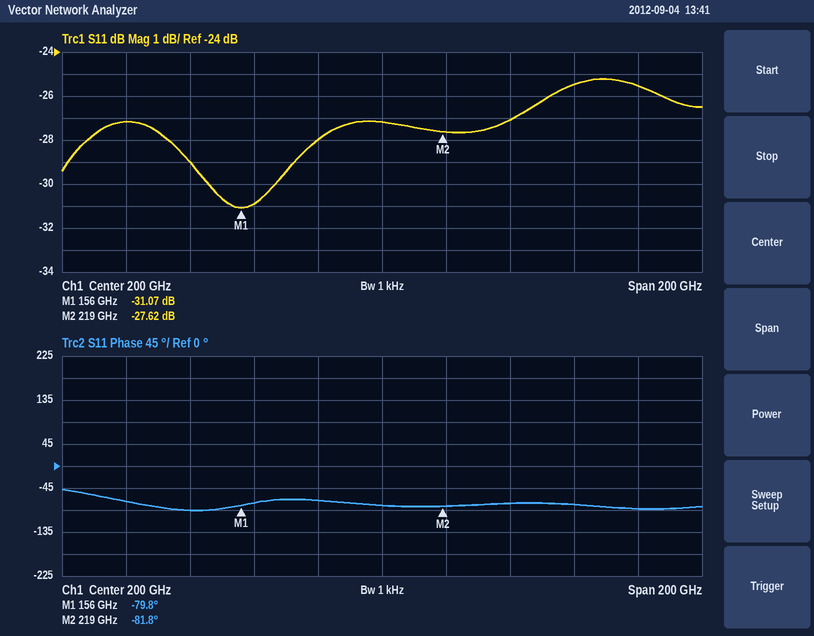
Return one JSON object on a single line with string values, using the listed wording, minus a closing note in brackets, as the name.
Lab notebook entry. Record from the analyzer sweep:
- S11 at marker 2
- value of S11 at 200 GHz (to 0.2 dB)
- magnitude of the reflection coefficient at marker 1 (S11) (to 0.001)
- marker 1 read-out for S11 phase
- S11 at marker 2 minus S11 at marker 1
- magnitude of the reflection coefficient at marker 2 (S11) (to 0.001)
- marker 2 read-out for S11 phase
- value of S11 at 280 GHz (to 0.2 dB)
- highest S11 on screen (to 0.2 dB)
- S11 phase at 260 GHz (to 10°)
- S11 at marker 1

{"S11 at marker 2": "-27.62 dB", "value of S11 at 200 GHz": "-27.2 dB", "magnitude of the reflection coefficient at marker 1 (S11)": "0.028", "marker 1 read-out for S11 phase": "-79.8°", "S11 at marker 2 minus S11 at marker 1": "3.45 dB", "magnitude of the reflection coefficient at marker 2 (S11)": "0.042", "marker 2 read-out for S11 phase": "-81.8°", "value of S11 at 280 GHz": "-25.6 dB", "highest S11 on screen": "-25.2 dB", "S11 phase at 260 GHz": "-80°", "S11 at marker 1": "-31.07 dB"}
